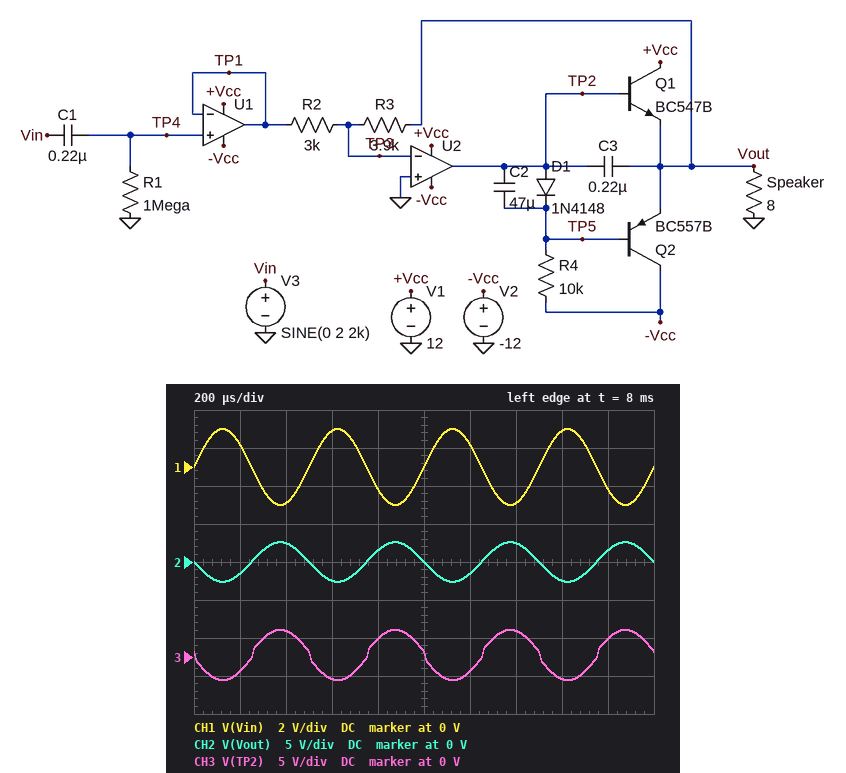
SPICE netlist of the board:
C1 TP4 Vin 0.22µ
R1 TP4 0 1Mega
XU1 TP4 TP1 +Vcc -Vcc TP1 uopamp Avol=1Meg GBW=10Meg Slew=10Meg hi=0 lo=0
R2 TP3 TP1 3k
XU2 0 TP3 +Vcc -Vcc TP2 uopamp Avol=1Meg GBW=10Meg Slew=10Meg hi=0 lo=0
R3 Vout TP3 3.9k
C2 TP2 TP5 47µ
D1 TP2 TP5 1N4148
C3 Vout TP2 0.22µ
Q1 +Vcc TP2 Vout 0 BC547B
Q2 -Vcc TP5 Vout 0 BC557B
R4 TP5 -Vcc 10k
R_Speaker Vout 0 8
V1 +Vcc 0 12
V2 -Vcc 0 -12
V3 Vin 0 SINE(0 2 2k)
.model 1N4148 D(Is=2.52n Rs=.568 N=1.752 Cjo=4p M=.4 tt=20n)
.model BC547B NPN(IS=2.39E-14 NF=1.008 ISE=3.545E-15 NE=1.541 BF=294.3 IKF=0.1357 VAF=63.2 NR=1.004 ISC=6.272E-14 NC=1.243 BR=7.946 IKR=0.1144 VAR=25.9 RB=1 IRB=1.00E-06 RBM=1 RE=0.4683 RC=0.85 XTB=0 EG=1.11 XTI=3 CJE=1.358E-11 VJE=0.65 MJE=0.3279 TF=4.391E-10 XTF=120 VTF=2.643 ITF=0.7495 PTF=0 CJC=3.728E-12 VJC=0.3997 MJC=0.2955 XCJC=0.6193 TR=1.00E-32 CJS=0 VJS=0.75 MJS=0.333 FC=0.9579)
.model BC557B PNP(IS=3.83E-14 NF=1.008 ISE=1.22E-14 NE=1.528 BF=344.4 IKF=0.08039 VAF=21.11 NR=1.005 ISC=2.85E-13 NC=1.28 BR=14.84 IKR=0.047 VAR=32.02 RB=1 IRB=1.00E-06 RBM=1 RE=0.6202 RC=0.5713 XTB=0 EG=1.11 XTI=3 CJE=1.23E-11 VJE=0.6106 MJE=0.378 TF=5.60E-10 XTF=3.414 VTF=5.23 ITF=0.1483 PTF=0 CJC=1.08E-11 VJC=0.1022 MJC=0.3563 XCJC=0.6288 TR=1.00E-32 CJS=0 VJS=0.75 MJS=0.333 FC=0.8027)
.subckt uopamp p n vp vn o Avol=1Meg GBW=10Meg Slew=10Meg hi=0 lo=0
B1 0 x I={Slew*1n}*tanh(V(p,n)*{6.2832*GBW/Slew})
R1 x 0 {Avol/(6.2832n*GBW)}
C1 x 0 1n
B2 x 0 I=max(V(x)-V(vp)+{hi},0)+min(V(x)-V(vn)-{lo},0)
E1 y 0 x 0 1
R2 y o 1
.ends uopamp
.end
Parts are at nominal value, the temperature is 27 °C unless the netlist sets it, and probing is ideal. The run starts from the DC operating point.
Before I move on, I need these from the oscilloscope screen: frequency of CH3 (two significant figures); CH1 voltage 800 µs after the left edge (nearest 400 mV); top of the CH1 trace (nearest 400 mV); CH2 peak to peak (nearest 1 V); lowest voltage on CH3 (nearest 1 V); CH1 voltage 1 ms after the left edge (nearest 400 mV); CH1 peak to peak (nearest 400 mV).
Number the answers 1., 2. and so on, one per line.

1. 2.0 kHz
2. -1.2 V
3. 2.0 V
4. 5 V
5. -3 V
6. 0 V
7. 4.0 V
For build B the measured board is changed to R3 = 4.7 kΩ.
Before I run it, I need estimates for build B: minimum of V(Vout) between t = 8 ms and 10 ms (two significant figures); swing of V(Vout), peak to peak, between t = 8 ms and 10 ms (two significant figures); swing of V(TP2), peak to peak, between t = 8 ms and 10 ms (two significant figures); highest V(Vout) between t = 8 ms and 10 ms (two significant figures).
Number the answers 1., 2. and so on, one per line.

1. -3.1 V
2. 6.3 V
3. 7.8 V
4. 3.1 V
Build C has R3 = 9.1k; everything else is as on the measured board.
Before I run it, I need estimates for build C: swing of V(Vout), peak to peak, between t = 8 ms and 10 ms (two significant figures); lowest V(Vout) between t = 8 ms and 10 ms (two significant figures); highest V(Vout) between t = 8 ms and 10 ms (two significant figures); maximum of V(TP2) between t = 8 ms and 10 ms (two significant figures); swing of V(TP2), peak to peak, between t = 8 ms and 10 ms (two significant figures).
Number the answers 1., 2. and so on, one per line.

1. 12 V
2. -6.1 V
3. 6.1 V
4. 7.3 V
5. 15 V
